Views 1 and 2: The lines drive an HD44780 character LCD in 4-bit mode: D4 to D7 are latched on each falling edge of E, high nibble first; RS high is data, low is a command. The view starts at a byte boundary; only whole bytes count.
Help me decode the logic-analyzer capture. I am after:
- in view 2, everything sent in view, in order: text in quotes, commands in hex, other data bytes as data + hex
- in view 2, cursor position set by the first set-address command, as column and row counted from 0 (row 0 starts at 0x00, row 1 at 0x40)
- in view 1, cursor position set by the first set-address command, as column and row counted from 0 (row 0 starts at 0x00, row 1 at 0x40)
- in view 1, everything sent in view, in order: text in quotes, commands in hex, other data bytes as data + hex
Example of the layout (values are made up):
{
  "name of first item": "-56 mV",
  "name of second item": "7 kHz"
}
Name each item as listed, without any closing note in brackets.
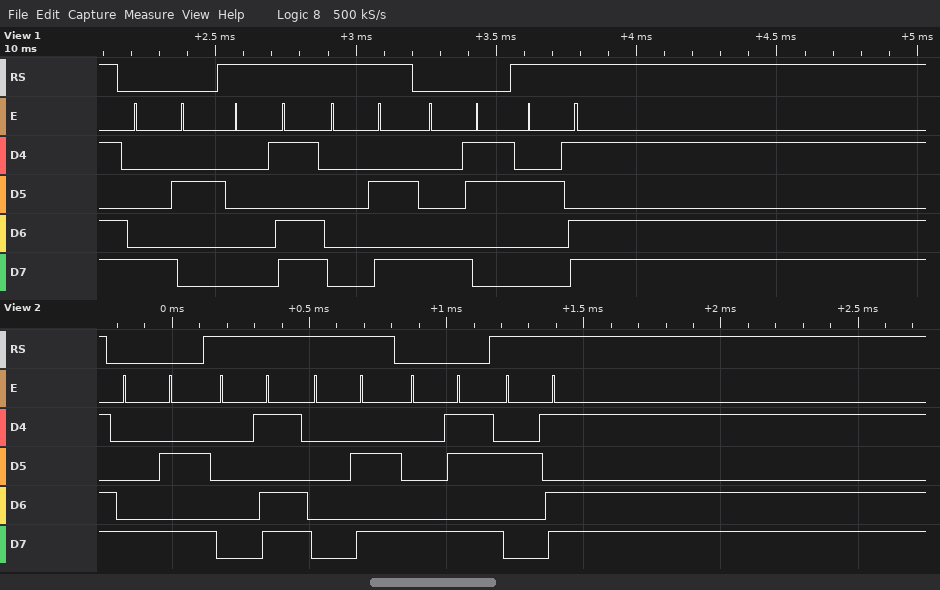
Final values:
{
  "in view 2, everything sent in view, in order: text in quotes, commands in hex, other data bytes as data + hex": "0x8A data 0D 0A 0x8B \"-\"",
  "in view 2, cursor position set by the first set-address command, as column and row counted from 0": "column 10, row 0",
  "in view 1, cursor position set by the first set-address command, as column and row counted from 0": "column 2, row 0",
  "in view 1, everything sent in view, in order: text in quotes, commands in hex, other data bytes as data + hex": "0x82 data 0D 0A 0x83 \"-\""
}
